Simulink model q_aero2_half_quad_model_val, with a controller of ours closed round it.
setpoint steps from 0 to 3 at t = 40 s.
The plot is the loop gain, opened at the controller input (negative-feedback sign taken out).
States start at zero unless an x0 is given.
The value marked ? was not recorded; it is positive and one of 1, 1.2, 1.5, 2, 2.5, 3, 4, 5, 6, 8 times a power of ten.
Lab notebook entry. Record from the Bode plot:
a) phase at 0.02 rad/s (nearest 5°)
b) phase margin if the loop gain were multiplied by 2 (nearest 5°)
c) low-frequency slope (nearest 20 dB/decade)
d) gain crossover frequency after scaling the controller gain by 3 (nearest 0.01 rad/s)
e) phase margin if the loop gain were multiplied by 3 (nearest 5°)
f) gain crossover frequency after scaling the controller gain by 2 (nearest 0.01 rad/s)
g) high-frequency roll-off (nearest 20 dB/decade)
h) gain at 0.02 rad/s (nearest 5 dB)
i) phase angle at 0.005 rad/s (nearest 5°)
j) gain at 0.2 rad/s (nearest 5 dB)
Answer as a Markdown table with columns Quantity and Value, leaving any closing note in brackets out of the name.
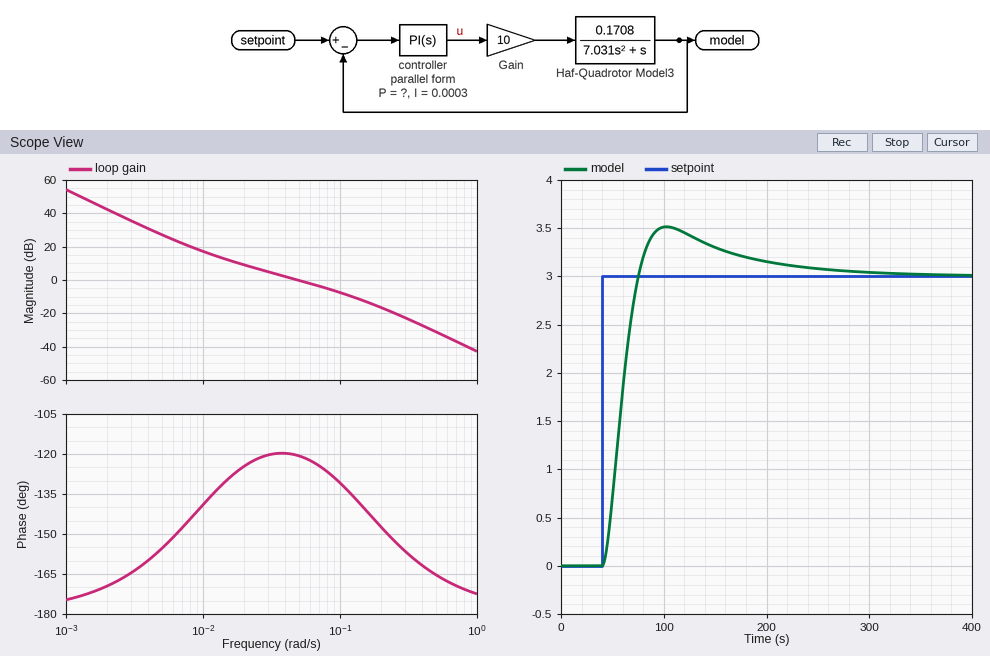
| Quantity | Value |
|---|---|
| phase at 0.02 rad/s | -125° |
| phase margin if the loop gain were multiplied by 2 | 50° |
| low-frequency slope | -40 dB/decade |
| gain crossover frequency after scaling the controller gain by 3 | 0.12 rad/s |
| phase margin if the loop gain were multiplied by 3 | 45° |
| gain crossover frequency after scaling the controller gain by 2 | 0.09 rad/s |
| high-frequency roll-off | -40 dB/decade |
| gain at 0.02 rad/s | 10 dB |
| phase angle at 0.005 rad/s | -155° |
| gain at 0.2 rad/s | -15 dB |
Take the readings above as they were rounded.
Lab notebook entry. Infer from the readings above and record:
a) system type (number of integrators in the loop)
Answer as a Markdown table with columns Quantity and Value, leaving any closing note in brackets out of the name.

| Quantity | Value |
|---|---|
| system type | 2 |
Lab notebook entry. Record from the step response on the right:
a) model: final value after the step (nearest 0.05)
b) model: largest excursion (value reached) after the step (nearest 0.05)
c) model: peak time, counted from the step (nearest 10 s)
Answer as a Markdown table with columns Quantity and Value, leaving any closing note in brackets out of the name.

| Quantity | Value |
|---|---|
| model: final value after the step | 3.00 |
| model: largest excursion (value reached) after the step | 3.50 |
| model: peak time, counted from the step | 60 s |
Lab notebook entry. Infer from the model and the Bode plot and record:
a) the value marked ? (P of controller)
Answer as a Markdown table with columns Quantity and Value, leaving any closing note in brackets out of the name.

| Quantity | Value |
|---|---|
| the value marked ? | 0.03 |
